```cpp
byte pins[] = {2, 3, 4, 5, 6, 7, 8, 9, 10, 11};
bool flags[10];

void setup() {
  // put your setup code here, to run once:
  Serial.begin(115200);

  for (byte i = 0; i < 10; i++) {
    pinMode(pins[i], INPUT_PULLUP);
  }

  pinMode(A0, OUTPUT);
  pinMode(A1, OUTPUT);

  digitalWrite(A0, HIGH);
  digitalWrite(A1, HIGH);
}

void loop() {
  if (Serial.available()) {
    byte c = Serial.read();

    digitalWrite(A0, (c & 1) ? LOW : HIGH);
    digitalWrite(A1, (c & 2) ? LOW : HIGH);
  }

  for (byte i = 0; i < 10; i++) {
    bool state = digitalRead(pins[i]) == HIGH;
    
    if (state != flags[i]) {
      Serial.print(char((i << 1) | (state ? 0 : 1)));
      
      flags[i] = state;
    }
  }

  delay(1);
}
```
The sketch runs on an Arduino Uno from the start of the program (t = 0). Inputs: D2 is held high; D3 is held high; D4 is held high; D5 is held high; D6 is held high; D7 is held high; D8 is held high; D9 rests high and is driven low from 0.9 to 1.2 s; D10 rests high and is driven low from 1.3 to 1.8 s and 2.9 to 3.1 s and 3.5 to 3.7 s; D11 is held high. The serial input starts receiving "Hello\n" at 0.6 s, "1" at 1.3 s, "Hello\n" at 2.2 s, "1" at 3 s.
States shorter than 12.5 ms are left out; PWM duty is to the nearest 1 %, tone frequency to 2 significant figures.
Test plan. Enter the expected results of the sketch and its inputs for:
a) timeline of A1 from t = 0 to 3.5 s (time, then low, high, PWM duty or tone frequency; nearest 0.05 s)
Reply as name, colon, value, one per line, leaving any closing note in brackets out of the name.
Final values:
timeline of A1 from t = 0 to 3.5 s: 0 s high; 0.6 s low; 1.3 s high; 2.2 s low; 3 s high
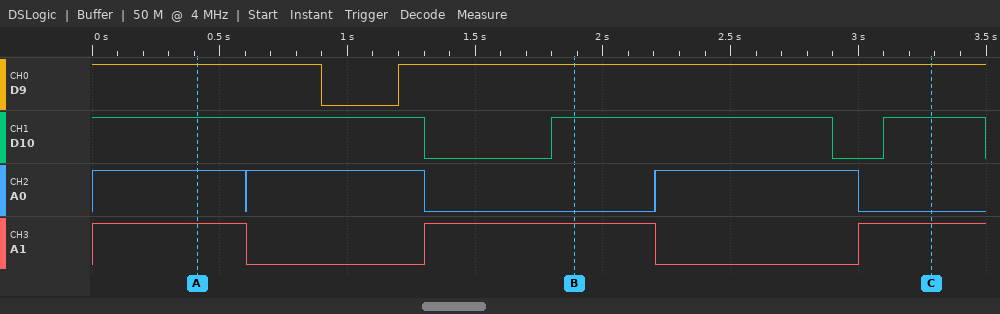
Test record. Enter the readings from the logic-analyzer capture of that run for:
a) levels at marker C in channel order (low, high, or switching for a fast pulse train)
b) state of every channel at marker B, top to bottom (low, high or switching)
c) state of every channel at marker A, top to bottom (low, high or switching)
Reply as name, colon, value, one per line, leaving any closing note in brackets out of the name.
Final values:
levels at marker C in channel order: D9 high, D10 high, A0 low, A1 high
state of every channel at marker B, top to bottom: D9 high, D10 high, A0 low, A1 high
state of every channel at marker A, top to bottom: D9 high, D10 high, A0 high, A1 high
